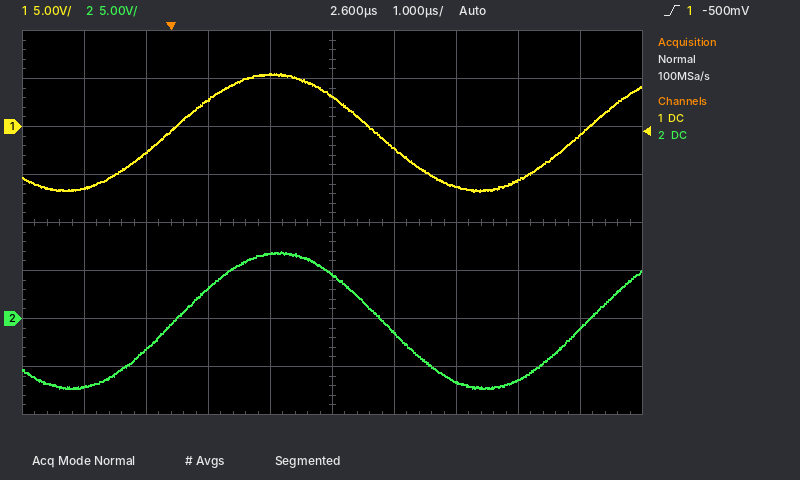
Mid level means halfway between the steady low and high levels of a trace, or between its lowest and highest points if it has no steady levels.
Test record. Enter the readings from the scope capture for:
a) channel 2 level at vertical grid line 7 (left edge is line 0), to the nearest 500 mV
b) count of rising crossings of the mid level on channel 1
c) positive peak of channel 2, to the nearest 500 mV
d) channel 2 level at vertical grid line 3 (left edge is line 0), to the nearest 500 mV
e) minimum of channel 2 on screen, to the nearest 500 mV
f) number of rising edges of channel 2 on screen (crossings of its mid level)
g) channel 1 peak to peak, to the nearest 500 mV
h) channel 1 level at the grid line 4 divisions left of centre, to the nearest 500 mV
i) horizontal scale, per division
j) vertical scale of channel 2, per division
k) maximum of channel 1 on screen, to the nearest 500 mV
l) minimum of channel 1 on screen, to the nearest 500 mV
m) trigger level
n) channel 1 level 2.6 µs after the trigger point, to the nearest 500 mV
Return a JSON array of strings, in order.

["-6.5 V", "2", "7.0 V", "3.0 V", "-7.5 V", "2", "12.5 V", "-6.5 V", "1 µs", "5 V", "5.5 V", "-7.0 V", "-500 mV", "3.0 V"]
